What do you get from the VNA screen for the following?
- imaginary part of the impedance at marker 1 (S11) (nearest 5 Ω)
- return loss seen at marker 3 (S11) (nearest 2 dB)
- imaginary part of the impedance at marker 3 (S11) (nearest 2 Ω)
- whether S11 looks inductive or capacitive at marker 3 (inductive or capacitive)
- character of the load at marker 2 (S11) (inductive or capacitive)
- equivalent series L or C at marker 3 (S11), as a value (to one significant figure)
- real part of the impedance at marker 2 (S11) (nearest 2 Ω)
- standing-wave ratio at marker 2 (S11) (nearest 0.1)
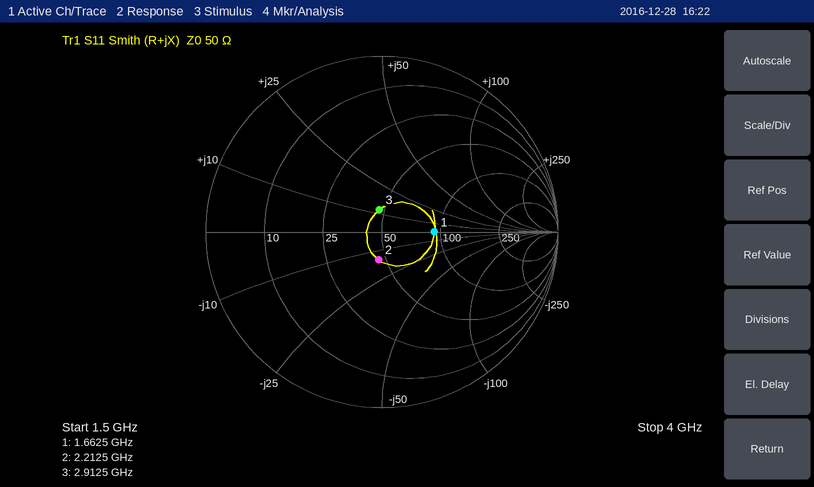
0 Ω
18 dB
+12 Ω
inductive
capacitive
700 pH
46 Ω
1.4
